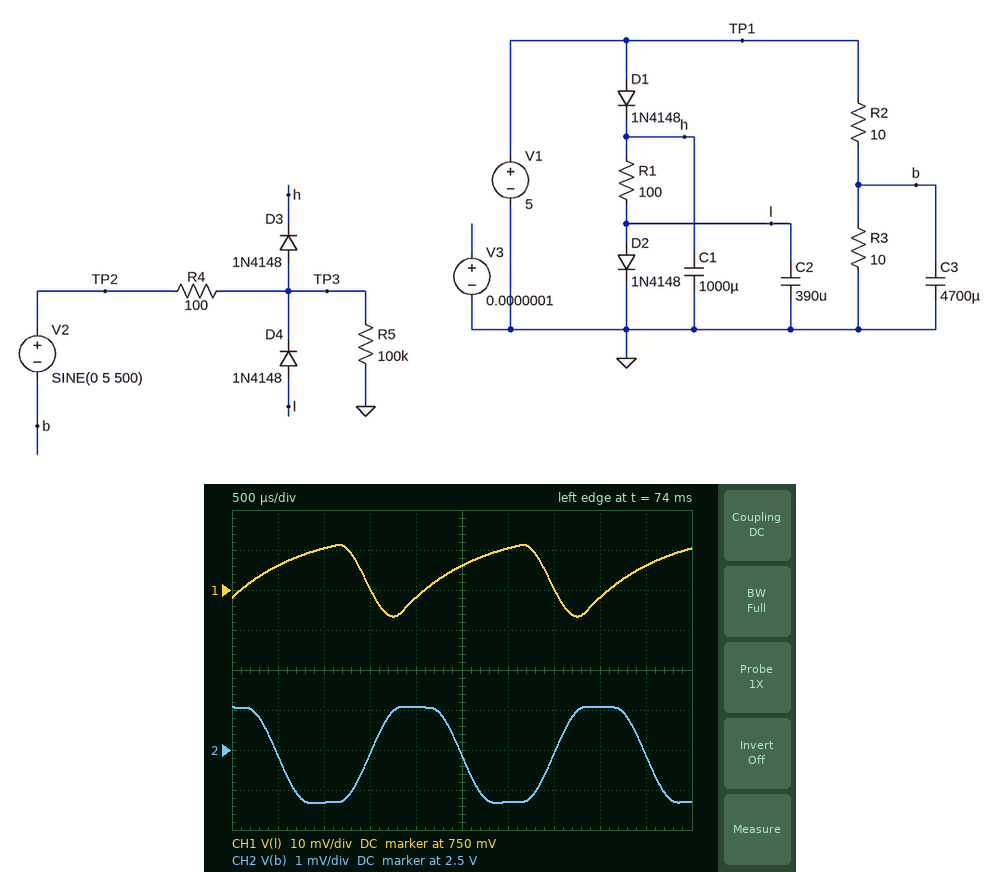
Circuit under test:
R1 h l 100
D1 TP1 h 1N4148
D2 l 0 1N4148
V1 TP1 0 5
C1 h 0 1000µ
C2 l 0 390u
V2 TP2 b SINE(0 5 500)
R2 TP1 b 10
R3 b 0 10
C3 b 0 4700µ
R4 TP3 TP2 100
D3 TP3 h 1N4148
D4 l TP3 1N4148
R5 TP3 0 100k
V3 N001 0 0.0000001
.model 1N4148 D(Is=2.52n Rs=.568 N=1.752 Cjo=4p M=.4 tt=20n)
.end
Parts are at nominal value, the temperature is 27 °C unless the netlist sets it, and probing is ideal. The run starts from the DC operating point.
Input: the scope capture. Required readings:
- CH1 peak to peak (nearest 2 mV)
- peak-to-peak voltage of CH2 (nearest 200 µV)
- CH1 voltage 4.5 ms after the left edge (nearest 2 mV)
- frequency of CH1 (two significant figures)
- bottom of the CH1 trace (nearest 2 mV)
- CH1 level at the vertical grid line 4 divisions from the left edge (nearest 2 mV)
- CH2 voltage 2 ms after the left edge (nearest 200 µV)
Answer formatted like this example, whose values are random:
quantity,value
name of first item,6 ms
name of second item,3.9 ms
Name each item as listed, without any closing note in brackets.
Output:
quantity,value
CH1 peak to peak,18 mV
peak-to-peak voltage of CH2,2.4 mV
CH1 voltage 4.5 ms after the left edge,756 mV
frequency of CH1,500 Hz
bottom of the CH1 trace,744 mV
CH1 level at the vertical grid line 4 divisions from the left edge,748 mV
CH2 voltage 2 ms after the left edge,2.5010 V
